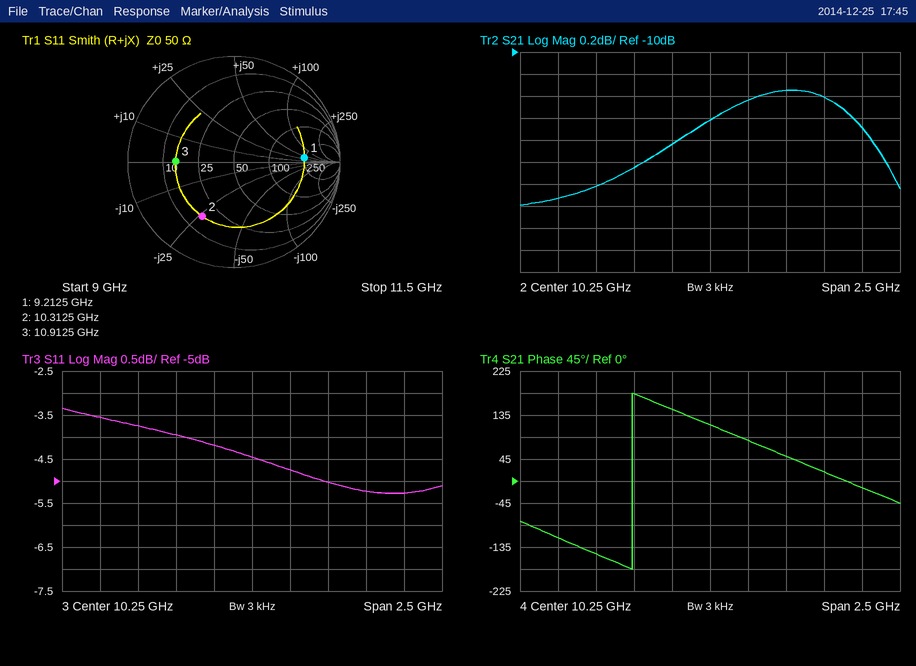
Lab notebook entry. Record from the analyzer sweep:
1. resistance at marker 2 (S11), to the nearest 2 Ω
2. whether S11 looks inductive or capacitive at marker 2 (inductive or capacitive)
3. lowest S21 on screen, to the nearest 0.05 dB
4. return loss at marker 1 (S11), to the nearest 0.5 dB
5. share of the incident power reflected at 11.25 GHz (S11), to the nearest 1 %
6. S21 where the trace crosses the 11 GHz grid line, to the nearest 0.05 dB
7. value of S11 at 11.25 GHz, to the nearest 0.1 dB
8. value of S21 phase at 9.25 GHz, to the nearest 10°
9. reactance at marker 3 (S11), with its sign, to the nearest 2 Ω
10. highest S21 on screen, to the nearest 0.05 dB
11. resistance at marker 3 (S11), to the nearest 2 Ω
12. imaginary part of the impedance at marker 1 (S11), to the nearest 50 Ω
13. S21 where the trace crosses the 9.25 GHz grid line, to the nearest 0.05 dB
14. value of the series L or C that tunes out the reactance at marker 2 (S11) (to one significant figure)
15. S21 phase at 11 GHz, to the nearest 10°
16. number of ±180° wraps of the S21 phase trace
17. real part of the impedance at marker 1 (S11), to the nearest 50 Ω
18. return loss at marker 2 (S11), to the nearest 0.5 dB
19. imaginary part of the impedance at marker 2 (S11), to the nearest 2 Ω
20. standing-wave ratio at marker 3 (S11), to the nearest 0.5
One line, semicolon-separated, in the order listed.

16 Ω; capacitive; -11.40 dB; 3.5 dB; 30 %; -10.40 dB; -5.3 dB; -120°; 0 Ω; -10.35 dB; 14 Ω; +50 Ω; -11.35 dB; 400 pH; 20°; 1; 250 Ω; 4.5 dB; -26 Ω; 3.5
